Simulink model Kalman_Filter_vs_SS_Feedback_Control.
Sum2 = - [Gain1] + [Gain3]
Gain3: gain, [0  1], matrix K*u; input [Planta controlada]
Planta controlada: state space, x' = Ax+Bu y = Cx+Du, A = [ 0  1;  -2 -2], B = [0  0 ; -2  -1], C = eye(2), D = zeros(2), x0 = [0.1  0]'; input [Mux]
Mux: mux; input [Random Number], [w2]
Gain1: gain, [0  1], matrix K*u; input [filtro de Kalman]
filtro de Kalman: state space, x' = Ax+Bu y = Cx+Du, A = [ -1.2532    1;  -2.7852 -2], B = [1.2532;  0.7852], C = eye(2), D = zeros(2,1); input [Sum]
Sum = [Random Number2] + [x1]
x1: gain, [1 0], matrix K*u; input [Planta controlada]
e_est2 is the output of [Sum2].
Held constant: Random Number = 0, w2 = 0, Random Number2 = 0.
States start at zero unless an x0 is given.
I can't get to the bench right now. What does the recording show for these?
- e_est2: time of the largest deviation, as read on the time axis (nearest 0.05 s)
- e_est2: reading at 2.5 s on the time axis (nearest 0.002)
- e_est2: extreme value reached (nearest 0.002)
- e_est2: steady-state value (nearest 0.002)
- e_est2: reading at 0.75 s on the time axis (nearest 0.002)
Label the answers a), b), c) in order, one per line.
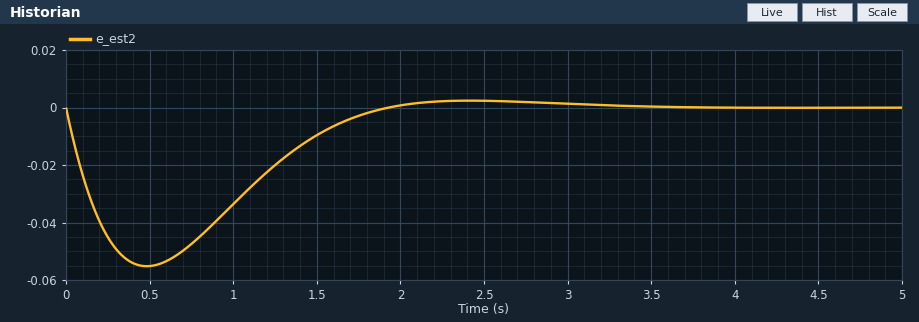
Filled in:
a) 0.50 s
b) 0.002
c) -0.056
d) 0.000
e) -0.048
